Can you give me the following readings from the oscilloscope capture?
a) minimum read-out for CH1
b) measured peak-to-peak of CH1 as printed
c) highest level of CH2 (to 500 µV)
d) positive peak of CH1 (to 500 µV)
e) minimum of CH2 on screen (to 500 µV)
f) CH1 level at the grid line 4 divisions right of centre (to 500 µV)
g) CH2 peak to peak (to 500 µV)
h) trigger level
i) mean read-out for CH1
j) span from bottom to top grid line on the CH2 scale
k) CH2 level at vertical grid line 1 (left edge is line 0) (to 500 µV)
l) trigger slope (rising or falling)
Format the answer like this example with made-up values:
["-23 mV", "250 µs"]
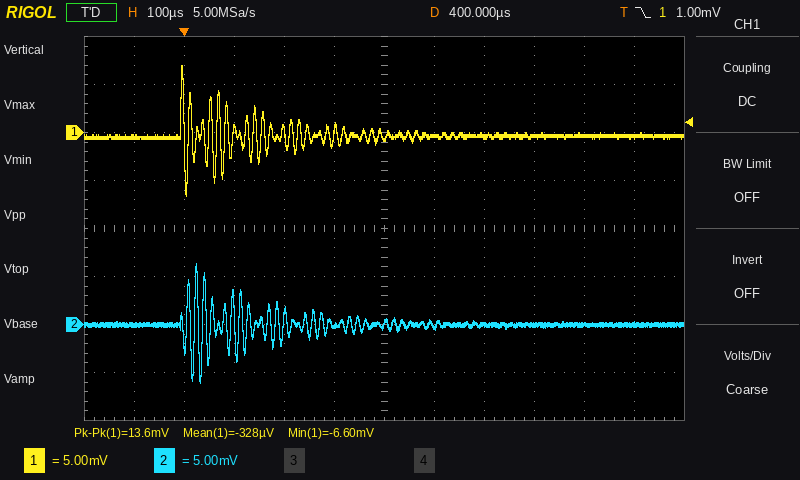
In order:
["-6.60 mV", "13.6 mV", "6.5 mV", "7.0 mV", "-6.0 mV", "-500 µV", "12.5 mV", "1.00 mV", "-328 µV", "40 mV", "0.0 mV", "falling"]
